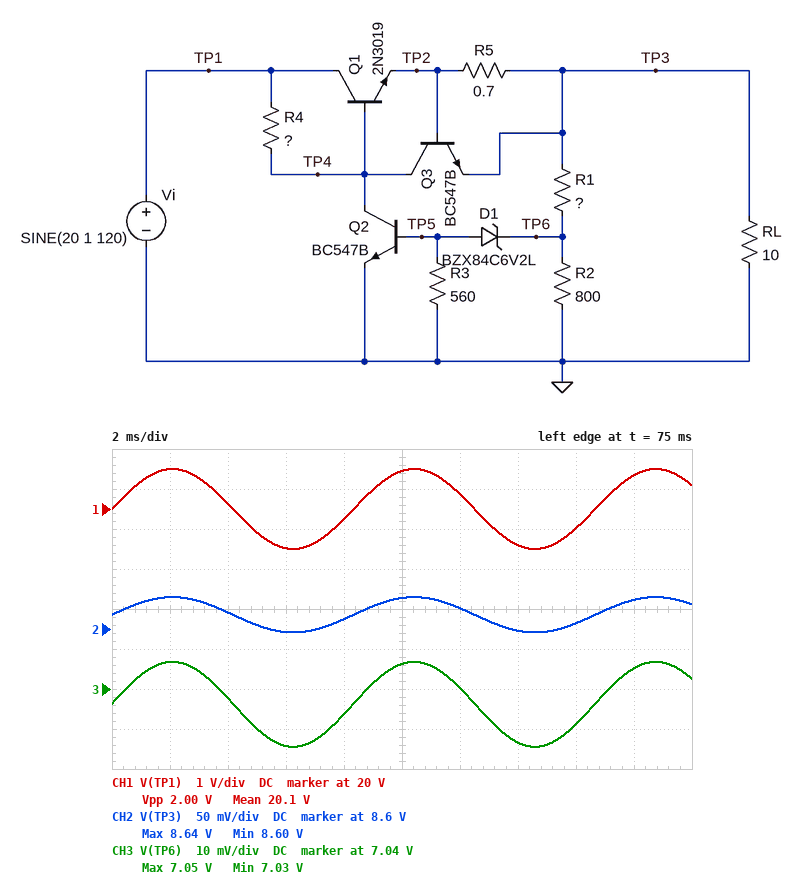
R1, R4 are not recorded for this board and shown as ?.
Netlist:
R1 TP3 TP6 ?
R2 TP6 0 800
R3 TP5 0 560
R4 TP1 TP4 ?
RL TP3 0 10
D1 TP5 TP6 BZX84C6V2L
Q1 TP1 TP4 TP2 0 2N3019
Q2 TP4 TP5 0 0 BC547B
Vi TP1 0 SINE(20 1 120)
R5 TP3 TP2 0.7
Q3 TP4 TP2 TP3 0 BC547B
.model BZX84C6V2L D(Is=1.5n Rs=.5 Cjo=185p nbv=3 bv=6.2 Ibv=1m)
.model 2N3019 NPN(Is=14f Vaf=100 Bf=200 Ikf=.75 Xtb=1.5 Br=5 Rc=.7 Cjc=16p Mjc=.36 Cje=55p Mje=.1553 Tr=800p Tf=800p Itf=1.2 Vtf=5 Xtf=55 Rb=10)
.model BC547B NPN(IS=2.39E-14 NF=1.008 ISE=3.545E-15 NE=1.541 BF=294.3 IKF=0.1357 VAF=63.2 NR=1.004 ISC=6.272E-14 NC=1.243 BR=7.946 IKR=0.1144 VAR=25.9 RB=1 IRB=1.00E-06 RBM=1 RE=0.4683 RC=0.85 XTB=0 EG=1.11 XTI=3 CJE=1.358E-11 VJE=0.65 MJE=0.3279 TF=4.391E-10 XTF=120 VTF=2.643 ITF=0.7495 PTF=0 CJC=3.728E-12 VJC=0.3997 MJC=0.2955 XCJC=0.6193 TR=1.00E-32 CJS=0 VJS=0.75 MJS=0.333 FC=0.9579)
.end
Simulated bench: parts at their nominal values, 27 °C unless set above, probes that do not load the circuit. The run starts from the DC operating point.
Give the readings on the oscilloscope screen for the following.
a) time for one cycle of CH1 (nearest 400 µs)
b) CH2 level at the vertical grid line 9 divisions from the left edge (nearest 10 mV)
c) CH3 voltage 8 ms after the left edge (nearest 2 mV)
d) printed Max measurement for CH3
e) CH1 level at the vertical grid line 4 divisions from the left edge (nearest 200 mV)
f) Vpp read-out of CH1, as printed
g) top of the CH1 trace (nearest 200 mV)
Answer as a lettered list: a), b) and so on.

a) 8.4 ms
b) 8.64 V
c) 7.034 V
d) 7.05 V
e) 19.8 V
f) 2.00 V
g) 21.0 V
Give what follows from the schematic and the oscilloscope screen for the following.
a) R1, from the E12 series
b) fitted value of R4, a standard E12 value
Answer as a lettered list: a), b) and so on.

a) 150 Ω
b) 120 Ω
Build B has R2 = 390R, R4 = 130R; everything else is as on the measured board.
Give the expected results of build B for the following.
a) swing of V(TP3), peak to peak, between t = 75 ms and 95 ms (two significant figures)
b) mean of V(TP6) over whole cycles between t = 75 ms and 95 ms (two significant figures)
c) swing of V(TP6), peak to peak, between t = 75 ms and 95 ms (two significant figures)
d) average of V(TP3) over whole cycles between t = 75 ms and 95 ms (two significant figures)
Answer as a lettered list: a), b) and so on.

a) 46 mV
b) 7.0 V
c) 22 mV
d) 9.9 V
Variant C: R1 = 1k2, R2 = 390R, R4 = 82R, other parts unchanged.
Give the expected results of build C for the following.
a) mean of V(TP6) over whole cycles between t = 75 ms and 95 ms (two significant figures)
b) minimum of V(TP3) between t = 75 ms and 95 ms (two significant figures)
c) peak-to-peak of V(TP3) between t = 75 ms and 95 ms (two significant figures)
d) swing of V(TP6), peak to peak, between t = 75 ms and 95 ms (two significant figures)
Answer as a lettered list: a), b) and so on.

a) 2.9 V
b) 12 V
c) 450 mV
d) 110 mV
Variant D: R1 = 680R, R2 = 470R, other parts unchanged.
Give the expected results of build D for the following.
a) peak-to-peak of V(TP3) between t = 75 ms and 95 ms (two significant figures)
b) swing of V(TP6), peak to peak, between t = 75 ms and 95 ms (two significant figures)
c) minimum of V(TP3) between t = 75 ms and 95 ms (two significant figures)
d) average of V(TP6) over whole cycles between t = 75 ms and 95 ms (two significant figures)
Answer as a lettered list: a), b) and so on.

a) 360 mV
b) 150 mV
c) 11 V
d) 4.6 V
